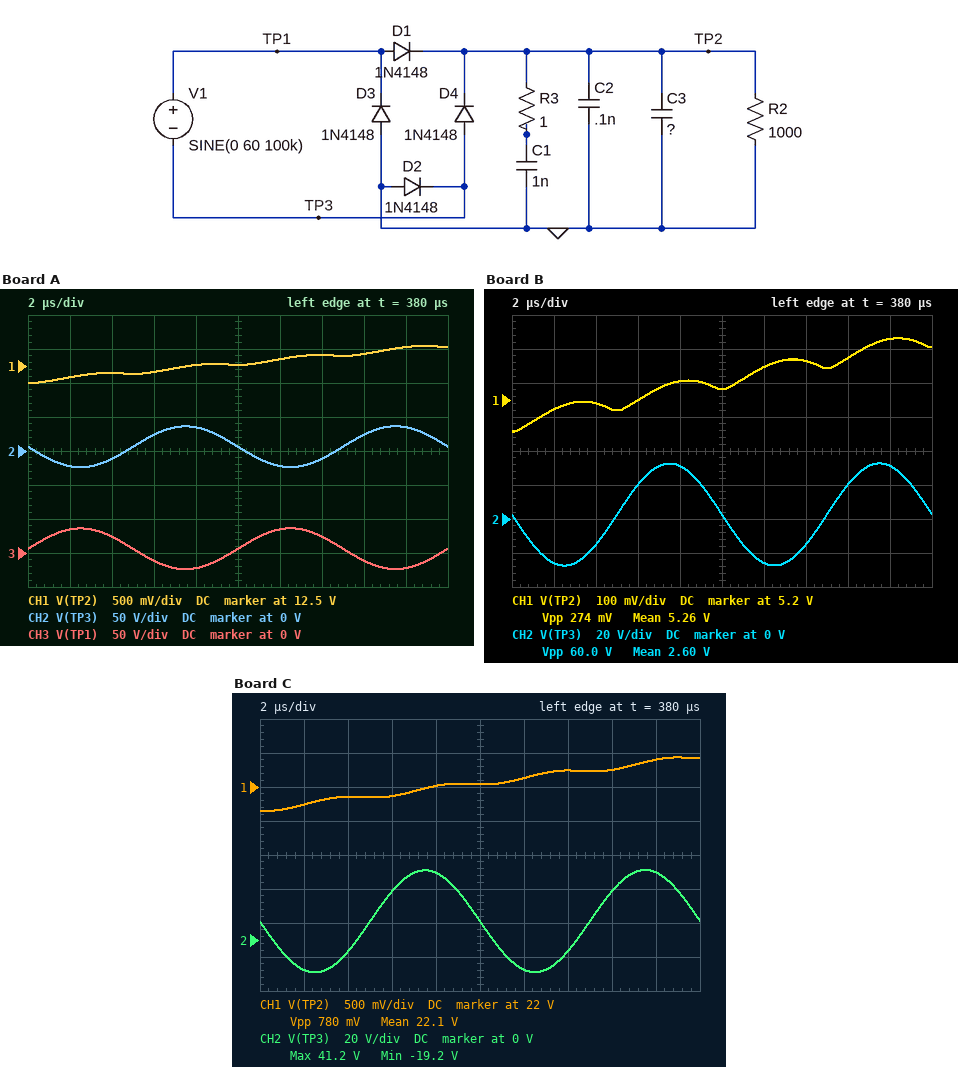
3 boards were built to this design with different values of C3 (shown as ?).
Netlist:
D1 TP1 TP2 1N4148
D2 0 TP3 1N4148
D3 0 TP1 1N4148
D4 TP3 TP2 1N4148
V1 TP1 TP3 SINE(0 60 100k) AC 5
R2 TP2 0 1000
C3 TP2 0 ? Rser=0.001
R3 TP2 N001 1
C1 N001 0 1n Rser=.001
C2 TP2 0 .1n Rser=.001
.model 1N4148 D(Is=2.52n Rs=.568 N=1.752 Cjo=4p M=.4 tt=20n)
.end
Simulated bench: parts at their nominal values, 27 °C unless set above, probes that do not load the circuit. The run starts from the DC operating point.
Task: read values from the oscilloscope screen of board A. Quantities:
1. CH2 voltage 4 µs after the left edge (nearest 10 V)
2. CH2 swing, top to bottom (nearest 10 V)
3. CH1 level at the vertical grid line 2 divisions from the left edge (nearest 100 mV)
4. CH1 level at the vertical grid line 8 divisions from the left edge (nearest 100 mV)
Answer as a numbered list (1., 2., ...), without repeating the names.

1. -10 V
2. 60 V
3. 12.4 V
4. 12.7 V
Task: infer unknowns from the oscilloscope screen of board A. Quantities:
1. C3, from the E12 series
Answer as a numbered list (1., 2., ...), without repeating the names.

1. 820 µF
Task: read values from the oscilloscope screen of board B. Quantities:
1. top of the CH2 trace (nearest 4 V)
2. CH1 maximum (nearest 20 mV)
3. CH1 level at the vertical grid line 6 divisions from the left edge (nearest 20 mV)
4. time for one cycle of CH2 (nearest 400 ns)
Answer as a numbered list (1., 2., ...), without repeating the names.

1. 32 V
2. 5.38 V
3. 5.30 V
4. 10.0 µs
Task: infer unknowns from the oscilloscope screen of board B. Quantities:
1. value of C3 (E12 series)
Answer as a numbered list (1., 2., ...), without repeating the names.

1. 2.2 mF
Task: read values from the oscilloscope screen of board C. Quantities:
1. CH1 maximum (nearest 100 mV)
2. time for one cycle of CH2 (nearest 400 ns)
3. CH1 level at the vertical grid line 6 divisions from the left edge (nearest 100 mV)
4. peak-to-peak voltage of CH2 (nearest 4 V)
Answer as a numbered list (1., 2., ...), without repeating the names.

1. 22.4 V
2. 10.0 µs
3. 22.1 V
4. 60 V
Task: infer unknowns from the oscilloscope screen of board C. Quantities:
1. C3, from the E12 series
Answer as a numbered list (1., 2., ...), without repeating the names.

1. 390 µF
